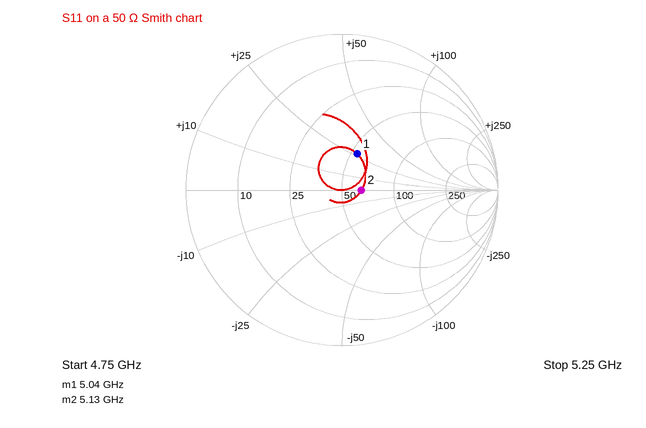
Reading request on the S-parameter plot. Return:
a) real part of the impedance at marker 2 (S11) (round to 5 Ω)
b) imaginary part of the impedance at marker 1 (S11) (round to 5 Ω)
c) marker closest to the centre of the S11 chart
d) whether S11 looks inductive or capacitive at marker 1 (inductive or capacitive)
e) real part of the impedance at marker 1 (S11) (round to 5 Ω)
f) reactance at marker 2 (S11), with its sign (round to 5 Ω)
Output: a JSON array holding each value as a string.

["65 Ω", "+25 Ω", "marker 2", "inductive", "55 Ω", "0 Ω"]
